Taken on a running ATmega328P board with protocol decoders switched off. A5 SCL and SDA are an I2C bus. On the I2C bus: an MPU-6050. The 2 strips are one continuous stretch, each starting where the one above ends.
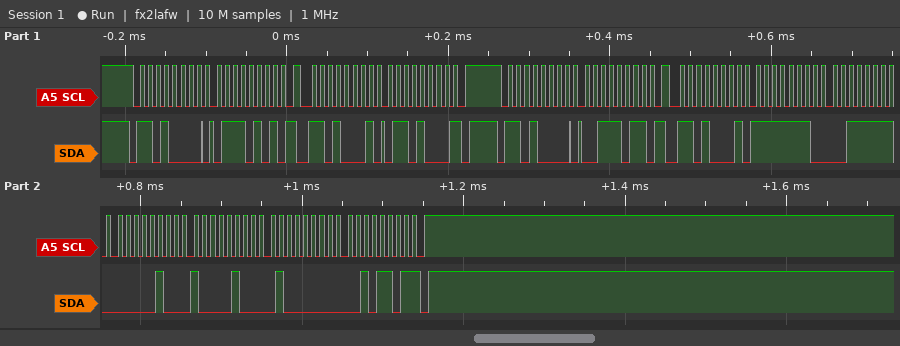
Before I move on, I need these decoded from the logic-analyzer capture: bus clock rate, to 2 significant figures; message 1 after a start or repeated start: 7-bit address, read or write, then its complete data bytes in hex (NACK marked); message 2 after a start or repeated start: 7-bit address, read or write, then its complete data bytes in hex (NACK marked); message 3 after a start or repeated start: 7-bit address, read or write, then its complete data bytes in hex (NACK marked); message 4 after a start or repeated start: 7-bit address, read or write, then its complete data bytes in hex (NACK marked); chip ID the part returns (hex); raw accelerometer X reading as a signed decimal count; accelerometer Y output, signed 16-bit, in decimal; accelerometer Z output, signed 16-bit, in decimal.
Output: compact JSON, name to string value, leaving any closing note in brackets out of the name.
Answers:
{"bus clock rate, to 2 significant figures": "100 kHz", "message 1 after a start or repeated start: 7-bit address, read or write, then its complete data bytes in hex": "0x68 write: 75", "message 2 after a start or repeated start: 7-bit address, read or write, then its complete data bytes in hex": "0x68 read: 68 NACK", "message 3 after a start or repeated start: 7-bit address, read or write, then its complete data bytes in hex": "0x68 write: 3B", "message 4 after a start or repeated start: 7-bit address, read or write, then its complete data bytes in hex": "0x68 read: FE 3F 04 84 40 2D NACK", "chip ID the part returns": "0x68", "raw accelerometer X reading as a signed decimal count": "-449", "accelerometer Y output, signed 16-bit, in decimal": "1156", "accelerometer Z output, signed 16-bit, in decimal": "16429"}
